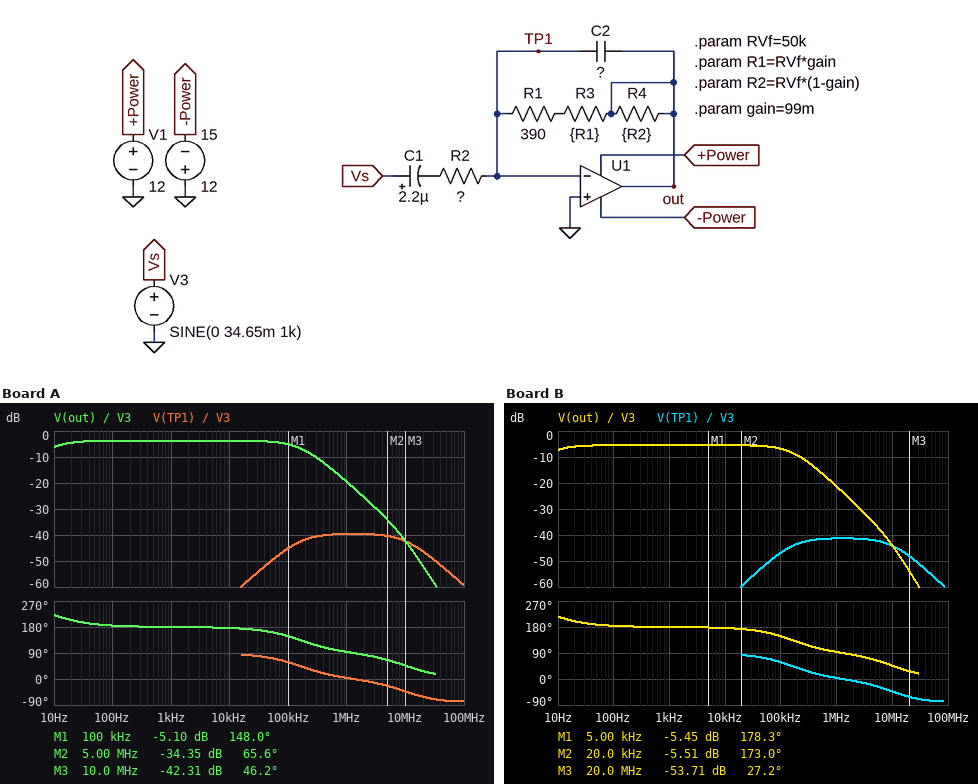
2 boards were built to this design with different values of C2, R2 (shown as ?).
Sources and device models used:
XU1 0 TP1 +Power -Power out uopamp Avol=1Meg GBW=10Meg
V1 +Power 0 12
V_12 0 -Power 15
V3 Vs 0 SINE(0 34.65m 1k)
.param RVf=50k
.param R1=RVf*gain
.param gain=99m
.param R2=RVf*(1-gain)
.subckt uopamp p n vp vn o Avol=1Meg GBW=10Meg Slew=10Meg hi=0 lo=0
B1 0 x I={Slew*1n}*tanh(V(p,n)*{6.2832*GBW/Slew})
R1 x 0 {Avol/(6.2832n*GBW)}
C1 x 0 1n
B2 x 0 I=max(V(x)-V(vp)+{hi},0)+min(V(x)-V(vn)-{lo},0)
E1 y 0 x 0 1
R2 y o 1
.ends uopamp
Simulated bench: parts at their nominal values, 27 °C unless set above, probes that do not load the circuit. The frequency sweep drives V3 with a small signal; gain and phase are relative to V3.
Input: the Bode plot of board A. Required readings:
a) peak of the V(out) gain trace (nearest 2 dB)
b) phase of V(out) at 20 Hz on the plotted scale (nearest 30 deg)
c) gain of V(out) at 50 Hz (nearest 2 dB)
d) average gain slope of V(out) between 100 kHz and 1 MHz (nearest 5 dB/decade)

-4 dB
210 deg
-4 dB
-15 dB/decade
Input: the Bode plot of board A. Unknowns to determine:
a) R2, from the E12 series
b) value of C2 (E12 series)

8.2 kΩ
180 pF
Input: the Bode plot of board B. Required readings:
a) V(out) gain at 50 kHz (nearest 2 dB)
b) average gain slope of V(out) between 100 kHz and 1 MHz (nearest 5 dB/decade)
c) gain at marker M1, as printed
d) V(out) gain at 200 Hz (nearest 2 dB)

-6 dB
-15 dB/decade
-5.45 dB
-6 dB
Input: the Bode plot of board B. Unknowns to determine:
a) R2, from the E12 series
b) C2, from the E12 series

10 kΩ
180 pF
